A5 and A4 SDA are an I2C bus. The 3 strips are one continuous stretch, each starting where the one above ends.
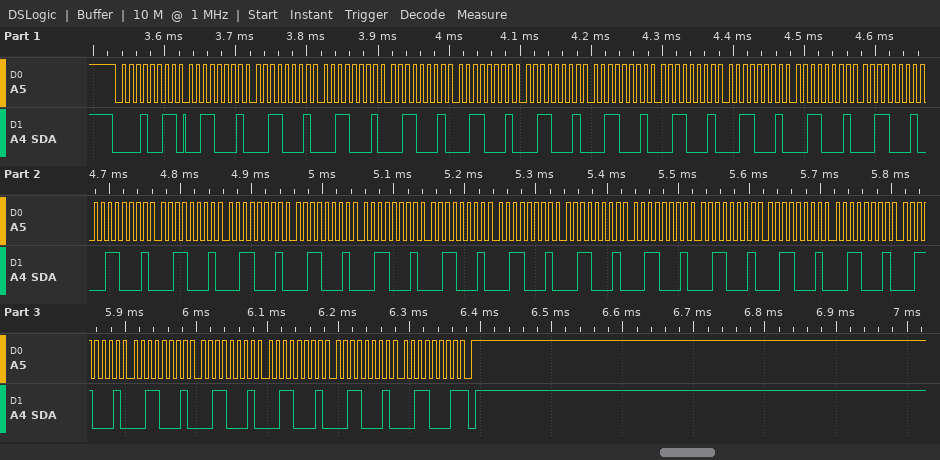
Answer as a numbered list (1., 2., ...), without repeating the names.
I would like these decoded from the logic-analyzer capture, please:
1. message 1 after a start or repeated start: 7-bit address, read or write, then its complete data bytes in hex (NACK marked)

1. 0x09 read: 31 31 31 31 31 31 31 31 31 31 31 31 31 31 31 31 31 31 31 31 31 31 31 31 31 31 31 31 31 NACK
